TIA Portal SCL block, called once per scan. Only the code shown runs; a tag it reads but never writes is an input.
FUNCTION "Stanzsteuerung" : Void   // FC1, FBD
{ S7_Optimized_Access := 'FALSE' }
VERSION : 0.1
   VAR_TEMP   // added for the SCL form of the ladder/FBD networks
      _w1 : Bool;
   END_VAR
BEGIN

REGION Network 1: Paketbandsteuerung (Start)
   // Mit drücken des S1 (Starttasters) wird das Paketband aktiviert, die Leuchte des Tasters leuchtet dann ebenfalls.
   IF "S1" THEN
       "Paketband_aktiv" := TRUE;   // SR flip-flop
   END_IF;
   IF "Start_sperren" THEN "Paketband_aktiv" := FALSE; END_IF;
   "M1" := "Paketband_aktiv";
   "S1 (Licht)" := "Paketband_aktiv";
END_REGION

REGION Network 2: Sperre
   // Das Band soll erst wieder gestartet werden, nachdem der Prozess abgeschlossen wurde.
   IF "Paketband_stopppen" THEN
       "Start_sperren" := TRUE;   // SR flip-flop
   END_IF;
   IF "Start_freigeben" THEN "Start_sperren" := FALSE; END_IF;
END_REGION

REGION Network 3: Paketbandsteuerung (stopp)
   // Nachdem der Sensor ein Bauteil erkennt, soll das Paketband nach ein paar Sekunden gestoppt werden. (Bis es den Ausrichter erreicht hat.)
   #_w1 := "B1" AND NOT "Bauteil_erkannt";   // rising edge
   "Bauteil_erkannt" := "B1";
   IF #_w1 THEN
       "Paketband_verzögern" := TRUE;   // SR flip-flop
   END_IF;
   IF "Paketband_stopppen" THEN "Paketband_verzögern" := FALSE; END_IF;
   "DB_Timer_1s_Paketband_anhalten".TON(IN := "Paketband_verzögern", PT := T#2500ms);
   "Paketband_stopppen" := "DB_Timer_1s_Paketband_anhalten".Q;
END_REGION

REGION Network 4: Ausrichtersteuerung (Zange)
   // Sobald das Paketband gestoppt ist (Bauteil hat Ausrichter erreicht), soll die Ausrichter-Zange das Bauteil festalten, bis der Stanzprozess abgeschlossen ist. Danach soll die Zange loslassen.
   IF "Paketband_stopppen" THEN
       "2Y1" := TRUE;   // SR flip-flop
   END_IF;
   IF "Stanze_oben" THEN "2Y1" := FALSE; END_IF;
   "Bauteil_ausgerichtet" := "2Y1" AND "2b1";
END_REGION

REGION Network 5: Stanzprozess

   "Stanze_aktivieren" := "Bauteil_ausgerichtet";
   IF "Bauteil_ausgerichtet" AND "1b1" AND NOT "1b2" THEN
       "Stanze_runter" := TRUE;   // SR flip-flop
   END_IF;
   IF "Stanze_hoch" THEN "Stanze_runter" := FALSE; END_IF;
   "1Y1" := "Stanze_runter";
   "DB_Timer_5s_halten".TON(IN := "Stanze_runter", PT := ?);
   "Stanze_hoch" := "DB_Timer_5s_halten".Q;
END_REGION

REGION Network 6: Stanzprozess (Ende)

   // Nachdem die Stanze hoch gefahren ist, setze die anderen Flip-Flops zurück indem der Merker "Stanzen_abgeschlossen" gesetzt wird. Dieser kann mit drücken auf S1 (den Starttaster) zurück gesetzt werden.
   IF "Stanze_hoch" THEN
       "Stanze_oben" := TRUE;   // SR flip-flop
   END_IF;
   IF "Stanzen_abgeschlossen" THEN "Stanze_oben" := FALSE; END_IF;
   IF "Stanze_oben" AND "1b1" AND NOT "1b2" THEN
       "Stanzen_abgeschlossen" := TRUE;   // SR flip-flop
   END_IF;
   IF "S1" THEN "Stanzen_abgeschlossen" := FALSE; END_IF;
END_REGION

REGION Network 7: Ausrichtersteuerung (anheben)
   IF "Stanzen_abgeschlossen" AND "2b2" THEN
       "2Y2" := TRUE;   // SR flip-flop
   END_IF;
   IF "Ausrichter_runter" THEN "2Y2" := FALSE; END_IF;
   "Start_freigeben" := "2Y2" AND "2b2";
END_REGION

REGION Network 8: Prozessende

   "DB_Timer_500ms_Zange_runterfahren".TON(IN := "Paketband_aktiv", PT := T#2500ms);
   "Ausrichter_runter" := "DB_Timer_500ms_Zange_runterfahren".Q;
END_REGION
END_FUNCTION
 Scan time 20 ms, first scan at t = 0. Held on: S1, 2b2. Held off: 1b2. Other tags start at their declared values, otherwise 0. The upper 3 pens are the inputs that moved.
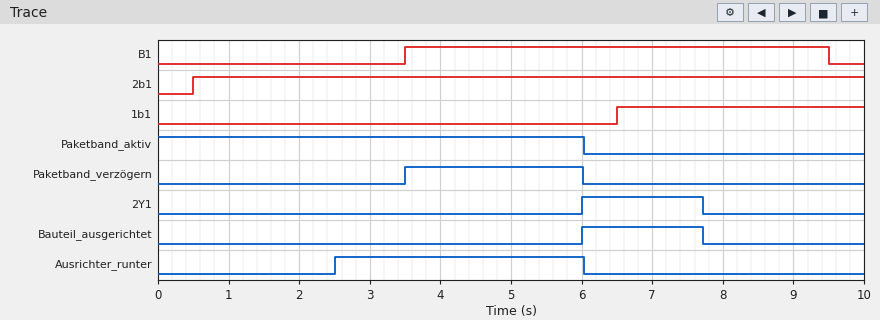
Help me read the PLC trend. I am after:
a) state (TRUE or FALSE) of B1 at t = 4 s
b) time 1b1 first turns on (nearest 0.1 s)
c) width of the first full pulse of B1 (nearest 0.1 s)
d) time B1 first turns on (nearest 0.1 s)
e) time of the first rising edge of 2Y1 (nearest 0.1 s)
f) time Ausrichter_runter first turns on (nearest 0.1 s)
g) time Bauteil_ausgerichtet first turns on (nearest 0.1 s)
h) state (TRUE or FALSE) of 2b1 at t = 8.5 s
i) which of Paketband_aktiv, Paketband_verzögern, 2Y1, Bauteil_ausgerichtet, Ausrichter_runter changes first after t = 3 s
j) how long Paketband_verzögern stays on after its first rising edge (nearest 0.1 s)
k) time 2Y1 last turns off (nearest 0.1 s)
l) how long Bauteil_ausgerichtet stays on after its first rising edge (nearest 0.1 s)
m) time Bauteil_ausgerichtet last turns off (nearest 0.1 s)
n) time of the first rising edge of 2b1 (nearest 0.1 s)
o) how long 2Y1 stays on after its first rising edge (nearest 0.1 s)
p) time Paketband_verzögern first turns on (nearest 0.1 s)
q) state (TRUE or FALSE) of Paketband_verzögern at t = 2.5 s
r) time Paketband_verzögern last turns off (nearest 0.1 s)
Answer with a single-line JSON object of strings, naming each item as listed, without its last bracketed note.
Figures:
{"state (TRUE or FALSE) of B1 at t = 4 s": "TRUE", "time 1b1 first turns on": "6.5 s", "width of the first full pulse of B1": "6.0 s", "time B1 first turns on": "3.5 s", "time of the first rising edge of 2Y1": "6.0 s", "time Ausrichter_runter first turns on": "2.5 s", "time Bauteil_ausgerichtet first turns on": "6.0 s", "state (TRUE or FALSE) of 2b1 at t = 8.5 s": "TRUE", "which of Paketband_aktiv, Paketband_verzögern, 2Y1, Bauteil_ausgerichtet, Ausrichter_runter changes first after t = 3 s": "Paketband_verzögern", "how long Paketband_verzögern stays on after its first rising edge": "2.5 s", "time 2Y1 last turns off": "7.7 s", "how long Bauteil_ausgerichtet stays on after its first rising edge": "1.7 s", "time Bauteil_ausgerichtet last turns off": "7.7 s", "time of the first rising edge of 2b1": "0.5 s", "how long 2Y1 stays on after its first rising edge": "1.7 s", "time Paketband_verzögern first turns on": "3.5 s", "state (TRUE or FALSE) of Paketband_verzögern at t = 2.5 s": "FALSE", "time Paketband_verzögern last turns off": "6.0 s"}
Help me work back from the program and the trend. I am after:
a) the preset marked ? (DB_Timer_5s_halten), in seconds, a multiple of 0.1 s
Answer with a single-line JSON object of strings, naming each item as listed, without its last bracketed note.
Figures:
{"the preset marked ? (DB_Timer_5s_halten), in seconds, a multiple of 0.1 s": "1.2 s"}
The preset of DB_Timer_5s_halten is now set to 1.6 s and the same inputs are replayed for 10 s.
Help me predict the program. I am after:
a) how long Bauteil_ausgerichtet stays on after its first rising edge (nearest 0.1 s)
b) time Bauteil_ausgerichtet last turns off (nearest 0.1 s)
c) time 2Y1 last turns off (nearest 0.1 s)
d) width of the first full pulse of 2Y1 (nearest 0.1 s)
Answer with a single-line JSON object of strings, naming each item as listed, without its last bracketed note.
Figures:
{"how long Bauteil_ausgerichtet stays on after its first rising edge": "2.1 s", "time Bauteil_ausgerichtet last turns off": "8.1 s", "time 2Y1 last turns off": "8.1 s", "width of the first full pulse of 2Y1": "2.1 s"}
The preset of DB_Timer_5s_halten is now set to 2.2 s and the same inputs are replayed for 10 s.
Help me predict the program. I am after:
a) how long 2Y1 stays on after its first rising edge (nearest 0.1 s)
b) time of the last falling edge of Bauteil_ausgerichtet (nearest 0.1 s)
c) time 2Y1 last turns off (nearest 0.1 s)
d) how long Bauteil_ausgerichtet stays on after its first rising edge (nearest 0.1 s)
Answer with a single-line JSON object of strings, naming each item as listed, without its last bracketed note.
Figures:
{"how long 2Y1 stays on after its first rising edge": "2.7 s", "time of the last falling edge of Bauteil_ausgerichtet": "8.7 s", "time 2Y1 last turns off": "8.7 s", "how long Bauteil_ausgerichtet stays on after its first rising edge": "2.7 s"}
